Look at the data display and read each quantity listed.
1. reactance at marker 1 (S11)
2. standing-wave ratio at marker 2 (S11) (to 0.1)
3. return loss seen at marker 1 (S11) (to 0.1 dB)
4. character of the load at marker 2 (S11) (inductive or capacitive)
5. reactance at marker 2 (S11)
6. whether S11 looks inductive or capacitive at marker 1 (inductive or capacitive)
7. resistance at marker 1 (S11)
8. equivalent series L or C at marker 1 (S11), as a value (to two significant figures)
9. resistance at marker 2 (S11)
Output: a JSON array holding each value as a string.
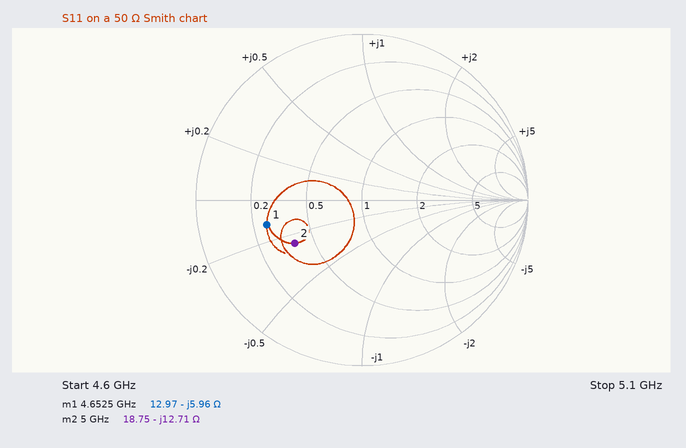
["-5.96 Ω", "2.9", "4.5 dB", "capacitive", "-12.71 Ω", "capacitive", "12.97 Ω", "5.7 pF", "18.75 Ω"]
